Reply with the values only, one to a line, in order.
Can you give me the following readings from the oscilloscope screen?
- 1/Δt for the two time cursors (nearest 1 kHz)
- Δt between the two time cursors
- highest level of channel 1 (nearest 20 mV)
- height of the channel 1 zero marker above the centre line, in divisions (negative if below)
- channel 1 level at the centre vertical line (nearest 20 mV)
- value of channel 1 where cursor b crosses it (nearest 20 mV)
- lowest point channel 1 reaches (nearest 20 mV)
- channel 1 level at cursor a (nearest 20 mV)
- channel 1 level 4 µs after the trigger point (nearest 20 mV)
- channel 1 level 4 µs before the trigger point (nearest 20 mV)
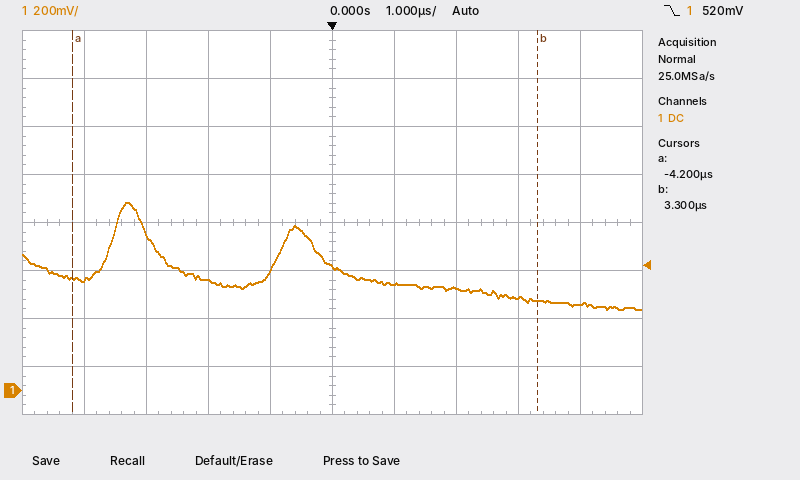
133 kHz
7.5 µs
780 mV
-3.5 div
520 mV
380 mV
340 mV
460 mV
360 mV
460 mV
